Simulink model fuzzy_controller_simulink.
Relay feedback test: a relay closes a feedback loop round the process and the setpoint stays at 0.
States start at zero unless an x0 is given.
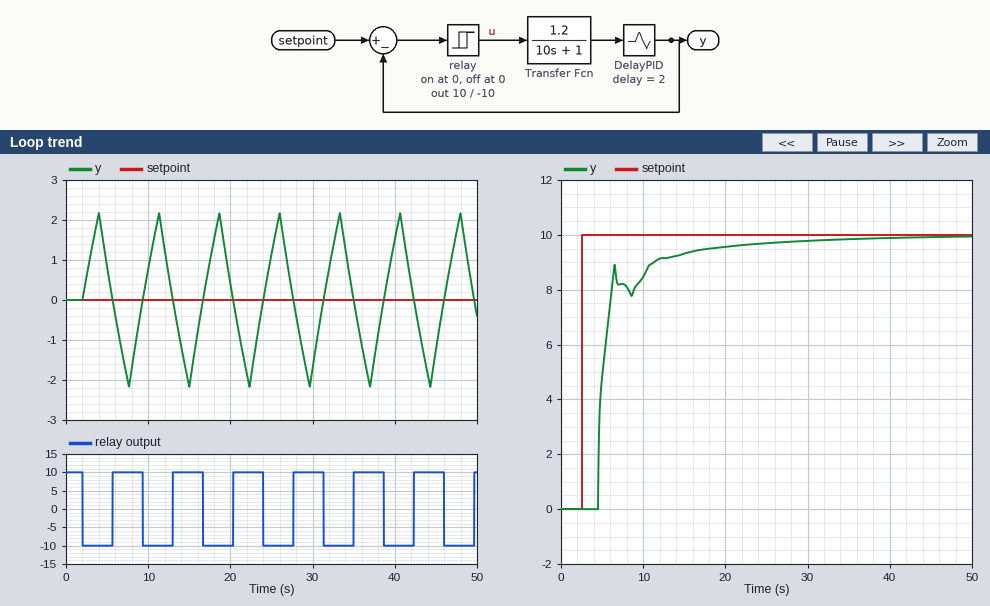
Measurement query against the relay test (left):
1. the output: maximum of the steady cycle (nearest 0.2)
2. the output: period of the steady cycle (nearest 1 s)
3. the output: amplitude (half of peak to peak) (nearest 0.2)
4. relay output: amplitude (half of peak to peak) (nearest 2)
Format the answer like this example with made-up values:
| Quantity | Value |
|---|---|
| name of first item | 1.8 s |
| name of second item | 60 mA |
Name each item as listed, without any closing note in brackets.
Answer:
| Quantity | Value |
|---|---|
| the output: maximum of the steady cycle | 2.2 |
| the output: period of the steady cycle | 7 s |
| the output: amplitude (half of peak to peak) | 2.2 |
| relay output: amplitude (half of peak to peak) | 10 |
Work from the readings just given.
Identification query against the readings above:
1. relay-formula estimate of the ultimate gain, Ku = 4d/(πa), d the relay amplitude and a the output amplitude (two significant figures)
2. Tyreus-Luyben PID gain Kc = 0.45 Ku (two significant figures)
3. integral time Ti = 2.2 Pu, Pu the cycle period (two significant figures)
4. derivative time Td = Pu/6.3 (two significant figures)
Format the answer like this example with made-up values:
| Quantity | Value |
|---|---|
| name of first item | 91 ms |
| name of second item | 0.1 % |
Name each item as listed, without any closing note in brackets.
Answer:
| Quantity | Value |
|---|---|
| relay-formula estimate of the ultimate gain, Ku = 4d/(πa), d the relay amplitude and a the output amplitude | 5.8 |
| Tyreus-Luyben PID gain Kc = 0.45 Ku | 2.6 |
| integral time Ti = 2.2 Pu, Pu the cycle period | 15 s |
| derivative time Td = Pu/6.3 | 1.1 s |
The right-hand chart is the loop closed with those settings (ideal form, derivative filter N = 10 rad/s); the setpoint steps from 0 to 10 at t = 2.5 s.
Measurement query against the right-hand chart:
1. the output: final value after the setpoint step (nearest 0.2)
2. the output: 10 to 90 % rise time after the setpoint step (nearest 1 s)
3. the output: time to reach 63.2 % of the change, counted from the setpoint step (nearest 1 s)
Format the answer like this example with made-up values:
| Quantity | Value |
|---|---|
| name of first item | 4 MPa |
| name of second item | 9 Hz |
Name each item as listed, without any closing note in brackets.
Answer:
| Quantity | Value |
|---|---|
| the output: final value after the setpoint step | 10.0 |
| the output: 10 to 90 % rise time after the setpoint step | 7 s |
| the output: time to reach 63.2 % of the change, counted from the setpoint step | 3 s |
